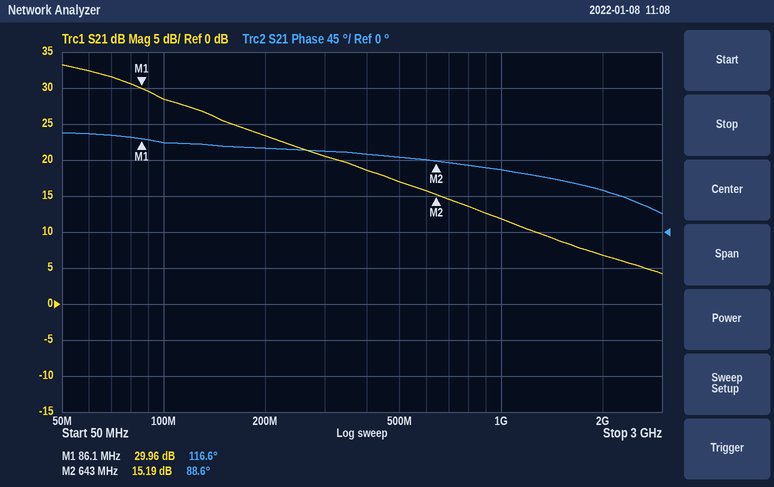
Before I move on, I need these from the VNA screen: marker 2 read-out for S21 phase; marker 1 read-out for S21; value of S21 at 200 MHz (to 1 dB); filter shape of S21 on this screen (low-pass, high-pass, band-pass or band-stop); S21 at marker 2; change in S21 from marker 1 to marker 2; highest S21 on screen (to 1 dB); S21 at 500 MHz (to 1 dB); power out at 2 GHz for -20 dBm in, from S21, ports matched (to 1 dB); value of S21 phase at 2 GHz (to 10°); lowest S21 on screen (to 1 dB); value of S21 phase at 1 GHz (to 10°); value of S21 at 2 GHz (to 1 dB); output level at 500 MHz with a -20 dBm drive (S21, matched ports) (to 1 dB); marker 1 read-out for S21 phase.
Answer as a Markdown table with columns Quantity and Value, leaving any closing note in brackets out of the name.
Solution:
| Quantity | Value |
|---|---|
| marker 2 read-out for S21 phase | 88.6° |
| marker 1 read-out for S21 | 29.96 dB |
| value of S21 at 200 MHz | 23 dB |
| filter shape of S21 on this screen | low-pass |
| S21 at marker 2 | 15.19 dB |
| change in S21 from marker 1 to marker 2 | -14.77 dB |
| highest S21 on screen | 33 dB |
| S21 at 500 MHz | 17 dB |
| power out at 2 GHz for -20 dBm in, from S21, ports matched | -13 dBm |
| value of S21 phase at 2 GHz | 50° |
| lowest S21 on screen | 4 dB |
| value of S21 phase at 1 GHz | 80° |
| value of S21 at 2 GHz | 7 dB |
| output level at 500 MHz with a -20 dBm drive (S21, matched ports) | -3 dBm |
| marker 1 read-out for S21 phase | 116.6° |
